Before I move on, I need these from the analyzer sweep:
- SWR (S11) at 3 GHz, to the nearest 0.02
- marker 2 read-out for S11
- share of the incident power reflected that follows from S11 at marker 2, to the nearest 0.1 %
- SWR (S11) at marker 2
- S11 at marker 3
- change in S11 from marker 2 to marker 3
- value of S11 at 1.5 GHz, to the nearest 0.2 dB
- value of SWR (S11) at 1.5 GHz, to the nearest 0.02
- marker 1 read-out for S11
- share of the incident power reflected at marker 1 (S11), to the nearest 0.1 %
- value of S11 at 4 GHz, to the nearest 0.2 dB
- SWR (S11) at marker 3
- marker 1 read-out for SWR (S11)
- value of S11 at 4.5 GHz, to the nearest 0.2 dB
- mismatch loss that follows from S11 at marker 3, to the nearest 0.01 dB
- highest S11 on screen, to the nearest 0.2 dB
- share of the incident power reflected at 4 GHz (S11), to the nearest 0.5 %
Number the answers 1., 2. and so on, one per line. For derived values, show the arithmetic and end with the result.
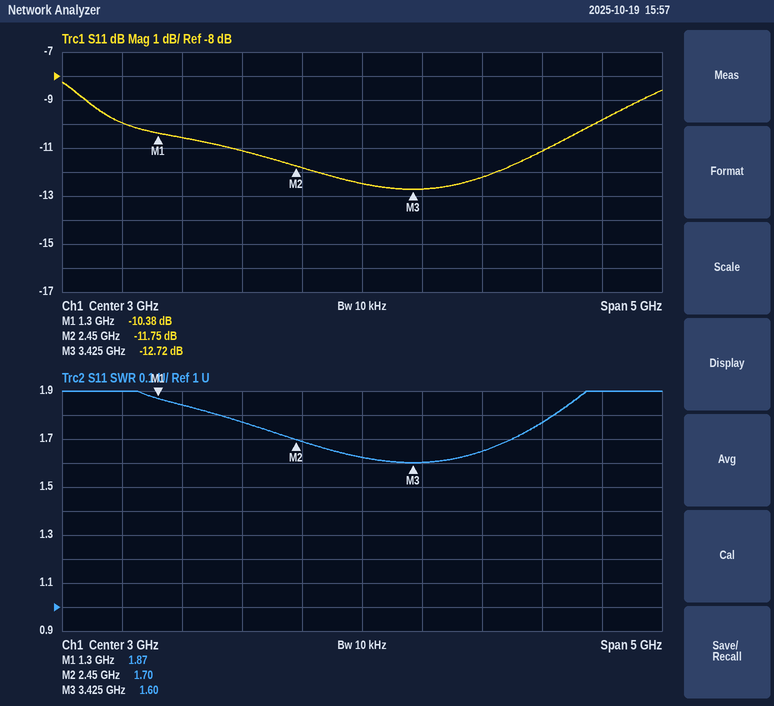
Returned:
1. 1.62
2. -11.75 dB
3. 10^(-11.75/10) ≈ 6.7 %
4. 1.70
5. -12.72 dB
6. -12.72 − (-11.75) = -0.97 dB
7. -10.6 dB
8. 1.84
9. -10.38 dB
10. 10^(-10.38/10) ≈ 9.2 %
11. -12.2 dB
12. 1.60
13. 1.87
14. -11.2 dB
15. −10 log10(1 − 10^(-12.72/10)) ≈ 0.24 dB
16. -8.2 dB
17. 10^(-12.2/10) ≈ 6.0 %
